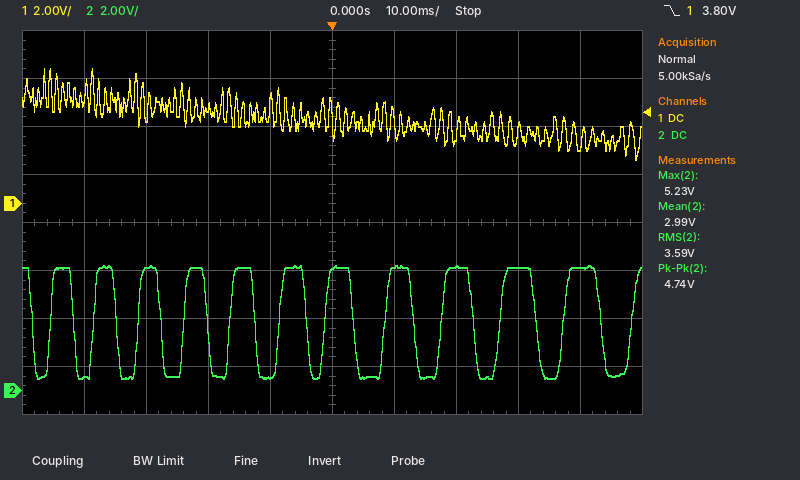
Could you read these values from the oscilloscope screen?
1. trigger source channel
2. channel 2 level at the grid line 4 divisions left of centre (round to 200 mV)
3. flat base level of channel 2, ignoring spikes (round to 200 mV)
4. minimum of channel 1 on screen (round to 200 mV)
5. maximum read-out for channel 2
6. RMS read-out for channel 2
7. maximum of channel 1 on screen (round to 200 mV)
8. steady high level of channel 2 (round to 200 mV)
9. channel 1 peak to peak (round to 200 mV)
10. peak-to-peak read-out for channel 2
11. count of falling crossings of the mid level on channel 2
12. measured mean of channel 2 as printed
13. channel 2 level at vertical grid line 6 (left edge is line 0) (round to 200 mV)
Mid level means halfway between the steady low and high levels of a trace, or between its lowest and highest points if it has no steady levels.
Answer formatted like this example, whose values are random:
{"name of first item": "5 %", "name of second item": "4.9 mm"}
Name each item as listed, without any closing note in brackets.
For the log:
{"trigger source channel": "channel 1", "channel 2 level at the grid line 4 divisions left of centre": "600 mV", "flat base level of channel 2, ignoring spikes": "600 mV", "minimum of channel 1 on screen": "1.8 V", "maximum read-out for channel 2": "5.23 V", "RMS read-out for channel 2": "3.59 V", "maximum of channel 1 on screen": "5.6 V", "steady high level of channel 2": "5.2 V", "channel 1 peak to peak": "3.8 V", "peak-to-peak read-out for channel 2": "4.74 V", "count of falling crossings of the mid level on channel 2": "12", "measured mean of channel 2 as printed": "2.99 V", "channel 2 level at vertical grid line 6 (left edge is line 0)": "5.2 V"}
